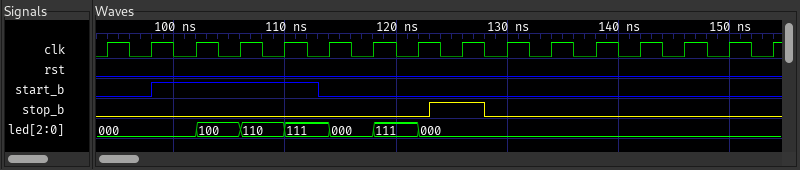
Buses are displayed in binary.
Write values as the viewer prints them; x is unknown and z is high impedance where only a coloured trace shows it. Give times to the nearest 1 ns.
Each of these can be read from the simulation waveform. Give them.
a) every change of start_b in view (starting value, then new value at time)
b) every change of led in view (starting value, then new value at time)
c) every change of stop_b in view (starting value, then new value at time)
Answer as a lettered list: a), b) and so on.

a) 0, 1 at 98 ns, 0 at 113 ns
b) 000, 100 at 102 ns, 110 at 106 ns, 111 at 110 ns, 000 at 114 ns, 111 at 118 ns, 000 at 122 ns
c) 0, 1 at 123 ns, 0 at 128 ns
